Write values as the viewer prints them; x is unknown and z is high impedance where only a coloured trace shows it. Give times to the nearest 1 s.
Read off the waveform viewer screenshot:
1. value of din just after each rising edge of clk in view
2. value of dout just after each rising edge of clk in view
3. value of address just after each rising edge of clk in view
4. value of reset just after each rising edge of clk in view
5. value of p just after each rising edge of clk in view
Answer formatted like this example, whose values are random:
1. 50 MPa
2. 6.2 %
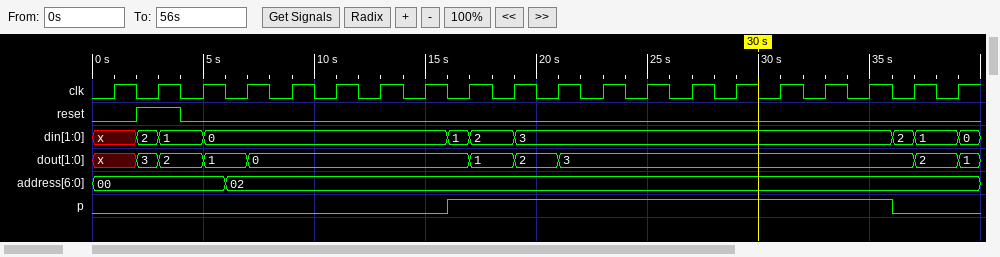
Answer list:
1. x, 1, 0, 0, 0, 0, 0, 0, 2, 3, 3, 3, 3, 3, 3, 3, 3, 3, 1, 0
2. x, 2, 1, 0, 0, 0, 0, 0, 1, 2, 3, 3, 3, 3, 3, 3, 3, 3, 2, 1
3. 00, 00, 00, 02, 02, 02, 02, 02, 02, 02, 02, 02, 02, 02, 02, 02, 02, 02, 02, 02
4. 0 1 0 0 0 0 0 0 0 0 0 0 0 0 0 0 0 0 0 0
5. 0 0 0 0 0 0 0 0 1 1 1 1 1 1 1 1 1 1 0 0
